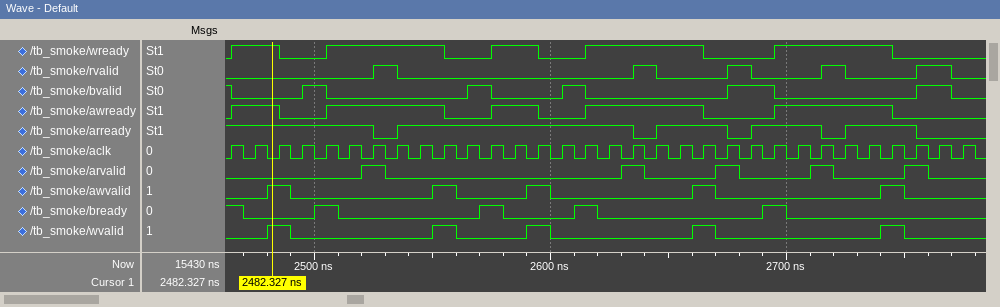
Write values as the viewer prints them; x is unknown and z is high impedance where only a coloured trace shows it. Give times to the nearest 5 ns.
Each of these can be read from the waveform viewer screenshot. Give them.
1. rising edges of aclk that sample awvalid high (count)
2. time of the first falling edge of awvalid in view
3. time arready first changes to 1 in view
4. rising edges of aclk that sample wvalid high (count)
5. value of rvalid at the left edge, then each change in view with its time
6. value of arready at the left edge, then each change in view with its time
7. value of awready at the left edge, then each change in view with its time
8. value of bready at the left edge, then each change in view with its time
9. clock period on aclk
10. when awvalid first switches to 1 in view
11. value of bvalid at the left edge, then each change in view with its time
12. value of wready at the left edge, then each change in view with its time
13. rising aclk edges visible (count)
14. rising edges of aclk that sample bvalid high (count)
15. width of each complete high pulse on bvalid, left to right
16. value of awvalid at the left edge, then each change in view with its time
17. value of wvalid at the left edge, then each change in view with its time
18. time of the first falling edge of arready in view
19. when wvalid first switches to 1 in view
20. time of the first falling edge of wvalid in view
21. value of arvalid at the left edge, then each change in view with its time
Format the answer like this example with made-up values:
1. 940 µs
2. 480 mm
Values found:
1. 5
2. 2490 ns
3. 2535 ns
4. 5
5. 0, 1 at 2525 ns, 0 at 2535 ns, 1 at 2635 ns, 0 at 2645 ns, 1 at 2675 ns, 0 at 2685 ns, 1 at 2715 ns, 0 at 2725 ns, 1 at 2755 ns, 0 at 2770 ns
6. 1, 0 at 2525 ns, 1 at 2535 ns, 0 at 2635 ns, 1 at 2645 ns, 0 at 2675 ns, 1 at 2685 ns, 0 at 2715 ns, 1 at 2725 ns, 0 at 2755 ns
7. 0, 1 at 2465 ns, 0 at 2485 ns, 1 at 2505 ns, 0 at 2555 ns, 1 at 2575 ns, 0 at 2595 ns, 1 at 2615 ns, 0 at 2665 ns, 1 at 2695 ns, 0 at 2745 ns
8. 1, 0 at 2470 ns, 1 at 2500 ns, 0 at 2510 ns, 1 at 2570 ns, 0 at 2580 ns, 1 at 2610 ns, 0 at 2620 ns, 1 at 2690 ns, 0 at 2700 ns
9. 10 ns
10. 2480 ns
11. 1, 0 at 2465 ns, 1 at 2495 ns, 0 at 2505 ns, 1 at 2565 ns, 0 at 2575 ns, 1 at 2605 ns, 0 at 2615 ns, 1 at 2675 ns, 0 at 2695 ns, 1 at 2755 ns, 0 at 2770 ns
12. 0, 1 at 2465 ns, 0 at 2485 ns, 1 at 2505 ns, 0 at 2555 ns, 1 at 2575 ns, 0 at 2595 ns, 1 at 2615 ns, 0 at 2665 ns, 1 at 2695 ns, 0 at 2745 ns
13. 32
14. 7
15. 10 ns, 10 ns, 10 ns, 20 ns, 15 ns
16. 0, 1 at 2480 ns, 0 at 2490 ns, 1 at 2550 ns, 0 at 2560 ns, 1 at 2590 ns, 0 at 2600 ns, 1 at 2660 ns, 0 at 2670 ns, 1 at 2740 ns, 0 at 2750 ns
17. 0, 1 at 2480 ns, 0 at 2490 ns, 1 at 2550 ns, 0 at 2560 ns, 1 at 2590 ns, 0 at 2600 ns, 1 at 2660 ns, 0 at 2670 ns, 1 at 2740 ns, 0 at 2750 ns
18. 2525 ns
19. 2480 ns
20. 2490 ns
21. 0, 1 at 2520 ns, 0 at 2530 ns, 1 at 2630 ns, 0 at 2640 ns, 1 at 2670 ns, 0 at 2680 ns, 1 at 2710 ns, 0 at 2720 ns, 1 at 2750 ns, 0 at 2760 ns
